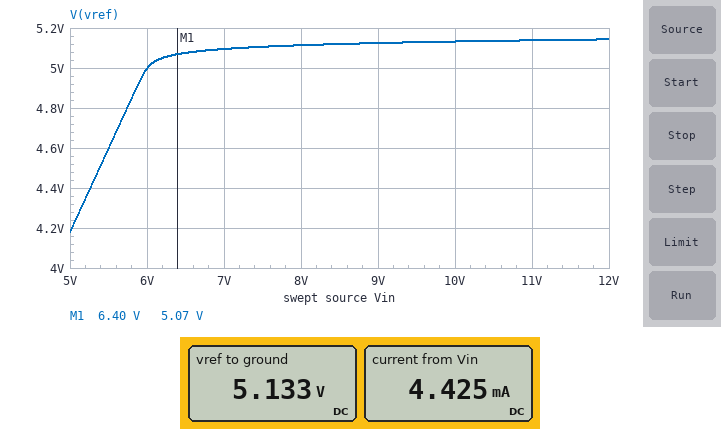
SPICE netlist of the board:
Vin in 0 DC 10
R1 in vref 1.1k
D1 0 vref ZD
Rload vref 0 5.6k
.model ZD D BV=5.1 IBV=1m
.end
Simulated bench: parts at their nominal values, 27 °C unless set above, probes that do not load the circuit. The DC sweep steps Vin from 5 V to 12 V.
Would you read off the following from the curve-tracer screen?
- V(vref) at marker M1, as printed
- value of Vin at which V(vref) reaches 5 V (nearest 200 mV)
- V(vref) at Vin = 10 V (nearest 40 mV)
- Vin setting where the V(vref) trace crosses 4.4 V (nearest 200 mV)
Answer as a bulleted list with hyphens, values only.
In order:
- 5.07 V
- 6.0 V
- 5.12 V
- 5.2 V
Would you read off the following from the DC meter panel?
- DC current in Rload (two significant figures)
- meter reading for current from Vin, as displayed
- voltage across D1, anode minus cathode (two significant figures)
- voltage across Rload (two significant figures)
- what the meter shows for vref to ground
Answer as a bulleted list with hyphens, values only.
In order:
- 920 µA
- 4.425 mA
- -5.1 V
- 5.1 V
- 5.133 V
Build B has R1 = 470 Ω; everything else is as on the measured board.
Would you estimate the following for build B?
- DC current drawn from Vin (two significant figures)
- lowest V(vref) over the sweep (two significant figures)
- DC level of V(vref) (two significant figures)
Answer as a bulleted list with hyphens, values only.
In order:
- 10 mA
- 4.6 V
- 5.2 V
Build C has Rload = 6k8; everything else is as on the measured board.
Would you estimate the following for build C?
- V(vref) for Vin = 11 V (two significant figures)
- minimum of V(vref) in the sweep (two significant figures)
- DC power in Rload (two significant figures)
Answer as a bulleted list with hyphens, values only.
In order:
- 5.1 V
- 4.3 V
- 3.9 mW
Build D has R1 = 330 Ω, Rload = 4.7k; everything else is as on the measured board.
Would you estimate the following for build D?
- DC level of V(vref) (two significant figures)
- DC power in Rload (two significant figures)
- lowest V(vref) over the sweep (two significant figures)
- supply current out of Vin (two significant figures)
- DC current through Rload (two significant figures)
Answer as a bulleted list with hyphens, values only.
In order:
- 5.2 V
- 5.7 mW
- 4.7 V
- 15 mA
- 1.1 mA
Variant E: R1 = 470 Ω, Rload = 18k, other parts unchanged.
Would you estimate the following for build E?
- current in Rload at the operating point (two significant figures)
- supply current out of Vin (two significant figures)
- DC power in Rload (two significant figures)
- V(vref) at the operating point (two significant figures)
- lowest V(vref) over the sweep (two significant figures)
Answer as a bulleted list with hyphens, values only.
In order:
- 290 µA
- 10 mA
- 1.5 mW
- 5.2 V
- 4.9 V
